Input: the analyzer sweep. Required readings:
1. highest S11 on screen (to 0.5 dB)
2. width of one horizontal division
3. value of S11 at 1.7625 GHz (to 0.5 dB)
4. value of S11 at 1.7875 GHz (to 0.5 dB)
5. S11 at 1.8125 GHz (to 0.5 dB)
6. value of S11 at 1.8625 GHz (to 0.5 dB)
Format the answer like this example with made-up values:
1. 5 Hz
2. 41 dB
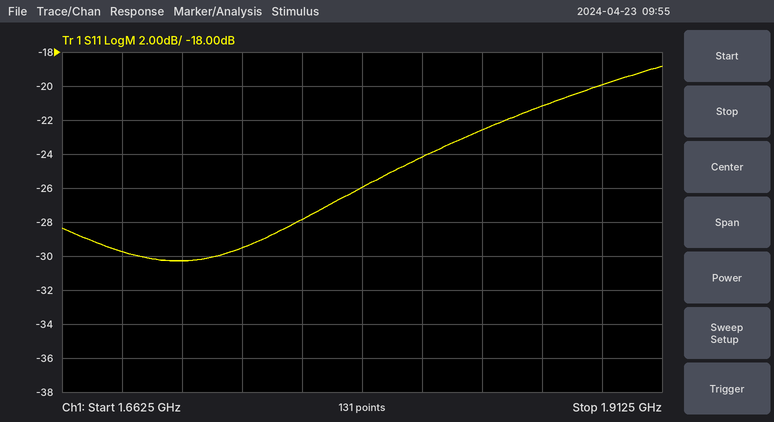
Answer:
1. -19.0 dB
2. 25 MHz
3. -28.0 dB
4. -26.0 dB
5. -24.0 dB
6. -21.0 dB
